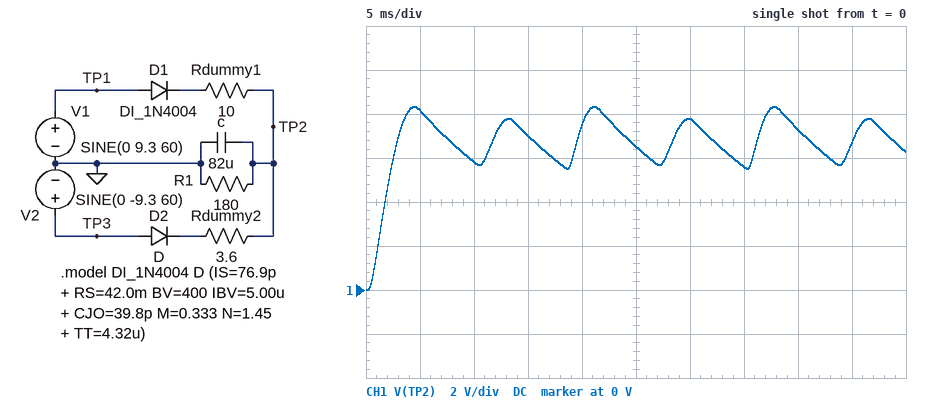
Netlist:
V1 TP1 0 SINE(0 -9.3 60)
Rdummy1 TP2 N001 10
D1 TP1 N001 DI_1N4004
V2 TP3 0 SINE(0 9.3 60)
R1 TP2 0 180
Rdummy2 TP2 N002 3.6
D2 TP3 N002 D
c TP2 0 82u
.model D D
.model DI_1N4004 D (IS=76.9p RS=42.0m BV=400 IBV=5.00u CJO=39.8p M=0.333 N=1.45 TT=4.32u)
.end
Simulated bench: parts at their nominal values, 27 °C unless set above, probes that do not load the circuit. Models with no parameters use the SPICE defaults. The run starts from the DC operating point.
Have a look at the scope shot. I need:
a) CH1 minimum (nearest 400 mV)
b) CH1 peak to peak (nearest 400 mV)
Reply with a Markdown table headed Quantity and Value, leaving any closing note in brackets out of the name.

| Quantity | Value |
|---|---|
| CH1 minimum | 0 V |
| CH1 peak to peak | 8.4 V |
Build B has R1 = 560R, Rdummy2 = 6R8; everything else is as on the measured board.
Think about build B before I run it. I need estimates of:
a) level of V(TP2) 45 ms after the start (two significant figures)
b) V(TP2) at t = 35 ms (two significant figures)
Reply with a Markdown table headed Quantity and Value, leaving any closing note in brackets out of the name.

| Quantity | Value |
|---|---|
| level of V(TP2) 45 ms after the start | 7.4 V |
| V(TP2) at t = 35 ms | 7.3 V |
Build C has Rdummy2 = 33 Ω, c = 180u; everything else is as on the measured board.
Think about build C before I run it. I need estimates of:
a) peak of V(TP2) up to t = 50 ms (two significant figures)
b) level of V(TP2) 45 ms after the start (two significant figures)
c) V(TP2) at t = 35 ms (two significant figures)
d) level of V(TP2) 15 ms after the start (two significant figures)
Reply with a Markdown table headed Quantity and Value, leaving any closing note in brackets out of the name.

| Quantity | Value |
|---|---|
| peak of V(TP2) up to t = 50 ms | 7.3 V |
| level of V(TP2) 45 ms after the start | 6.2 V |
| V(TP2) at t = 35 ms | 6.3 V |
| level of V(TP2) 15 ms after the start | 6.8 V |
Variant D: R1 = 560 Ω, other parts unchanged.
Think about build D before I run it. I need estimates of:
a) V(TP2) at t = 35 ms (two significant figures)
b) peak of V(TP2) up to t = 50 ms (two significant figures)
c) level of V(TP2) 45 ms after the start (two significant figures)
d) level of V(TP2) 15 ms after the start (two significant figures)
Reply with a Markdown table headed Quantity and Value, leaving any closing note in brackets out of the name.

| Quantity | Value |
|---|---|
| V(TP2) at t = 35 ms | 7.3 V |
| peak of V(TP2) up to t = 50 ms | 8.4 V |
| level of V(TP2) 45 ms after the start | 7.5 V |
| level of V(TP2) 15 ms after the start | 7.9 V |
